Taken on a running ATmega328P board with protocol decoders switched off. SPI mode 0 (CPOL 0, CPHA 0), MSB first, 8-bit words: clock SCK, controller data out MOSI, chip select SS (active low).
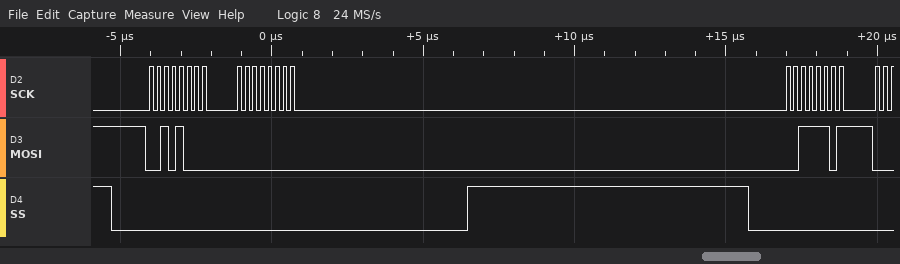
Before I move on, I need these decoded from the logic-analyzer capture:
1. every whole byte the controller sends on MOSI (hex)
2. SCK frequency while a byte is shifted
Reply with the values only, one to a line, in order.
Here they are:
0x28 0x00 0x3D
4 MHz
